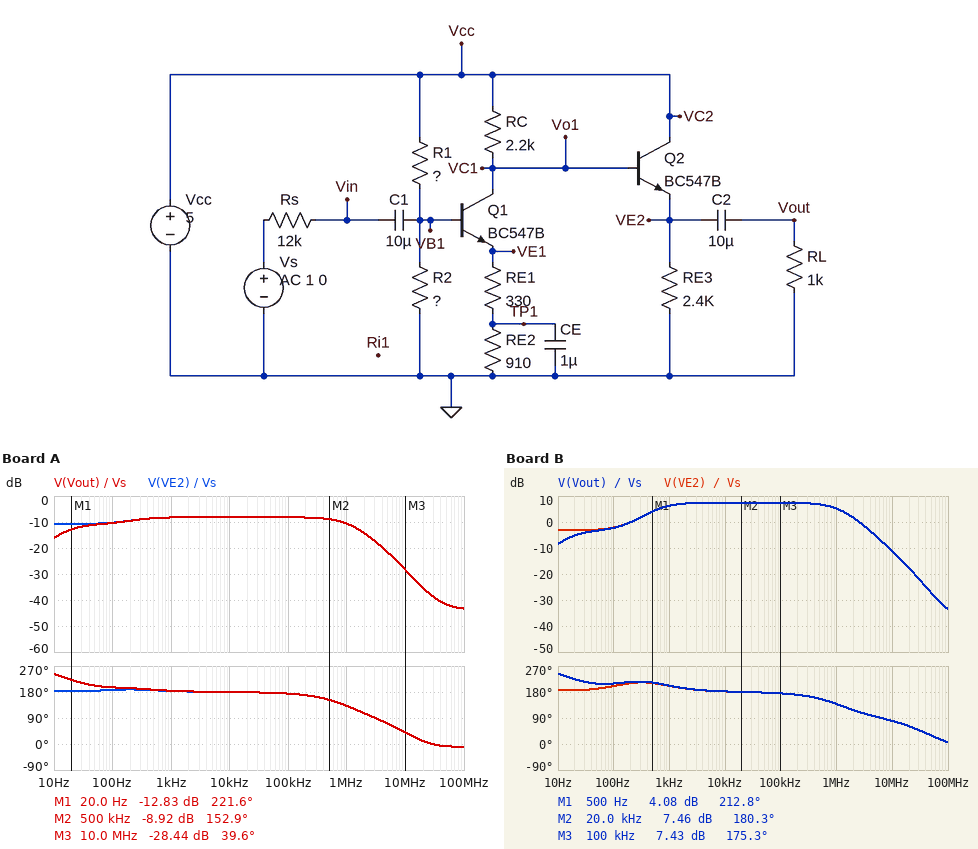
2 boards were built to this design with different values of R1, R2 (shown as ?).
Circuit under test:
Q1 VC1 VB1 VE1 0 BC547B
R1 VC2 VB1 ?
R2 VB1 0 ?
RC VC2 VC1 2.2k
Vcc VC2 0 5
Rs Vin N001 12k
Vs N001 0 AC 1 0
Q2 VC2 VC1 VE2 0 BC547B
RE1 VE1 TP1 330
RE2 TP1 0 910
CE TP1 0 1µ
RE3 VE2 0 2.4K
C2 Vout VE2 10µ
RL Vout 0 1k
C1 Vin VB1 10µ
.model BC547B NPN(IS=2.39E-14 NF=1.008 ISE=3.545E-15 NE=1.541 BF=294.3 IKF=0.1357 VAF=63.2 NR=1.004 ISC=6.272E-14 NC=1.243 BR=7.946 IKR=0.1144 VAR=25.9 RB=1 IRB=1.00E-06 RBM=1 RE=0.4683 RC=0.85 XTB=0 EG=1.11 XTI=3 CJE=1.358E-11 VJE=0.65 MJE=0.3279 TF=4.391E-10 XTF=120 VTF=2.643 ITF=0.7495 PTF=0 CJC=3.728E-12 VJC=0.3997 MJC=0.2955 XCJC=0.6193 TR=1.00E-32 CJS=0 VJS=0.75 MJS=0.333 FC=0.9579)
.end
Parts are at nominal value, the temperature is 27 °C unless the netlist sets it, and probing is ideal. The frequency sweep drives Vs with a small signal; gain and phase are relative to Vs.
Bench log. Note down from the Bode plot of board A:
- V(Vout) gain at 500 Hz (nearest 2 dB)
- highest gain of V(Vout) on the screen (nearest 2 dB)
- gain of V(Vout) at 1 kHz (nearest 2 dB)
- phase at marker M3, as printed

-8 dB
-8 dB
-8 dB
39.6 deg
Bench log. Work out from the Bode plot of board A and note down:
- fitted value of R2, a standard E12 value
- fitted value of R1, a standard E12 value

12 kΩ
100 kΩ
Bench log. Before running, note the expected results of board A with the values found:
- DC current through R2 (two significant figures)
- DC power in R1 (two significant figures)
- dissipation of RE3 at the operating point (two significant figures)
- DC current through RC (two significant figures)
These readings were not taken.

45 µA
200 µW
7.7 mW
18 µA
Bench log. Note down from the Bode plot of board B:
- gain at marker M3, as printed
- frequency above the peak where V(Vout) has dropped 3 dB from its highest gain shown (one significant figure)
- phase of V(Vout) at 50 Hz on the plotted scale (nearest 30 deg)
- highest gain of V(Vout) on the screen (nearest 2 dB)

7.43 dB
1 MHz
210 deg
8 dB
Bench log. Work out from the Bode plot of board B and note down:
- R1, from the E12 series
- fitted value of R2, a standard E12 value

22 kΩ
15 kΩ
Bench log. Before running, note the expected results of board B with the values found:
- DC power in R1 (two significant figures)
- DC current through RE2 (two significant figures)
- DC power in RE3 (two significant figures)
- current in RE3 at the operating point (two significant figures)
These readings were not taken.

410 µW
1.1 mA
1.6 mW
820 µA
